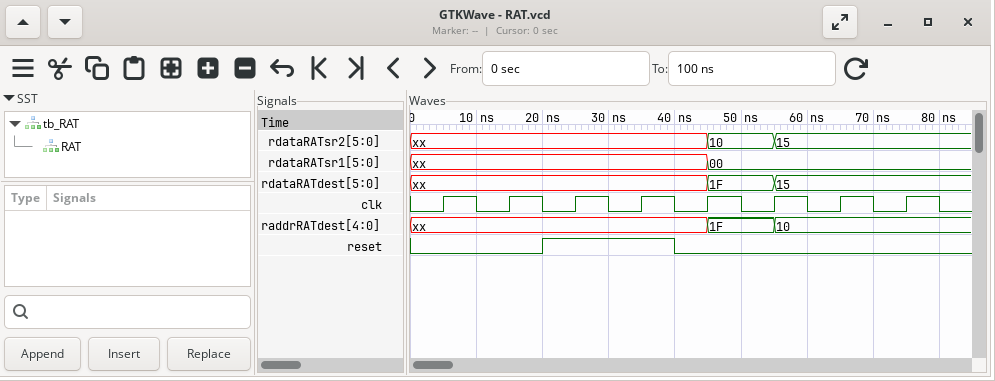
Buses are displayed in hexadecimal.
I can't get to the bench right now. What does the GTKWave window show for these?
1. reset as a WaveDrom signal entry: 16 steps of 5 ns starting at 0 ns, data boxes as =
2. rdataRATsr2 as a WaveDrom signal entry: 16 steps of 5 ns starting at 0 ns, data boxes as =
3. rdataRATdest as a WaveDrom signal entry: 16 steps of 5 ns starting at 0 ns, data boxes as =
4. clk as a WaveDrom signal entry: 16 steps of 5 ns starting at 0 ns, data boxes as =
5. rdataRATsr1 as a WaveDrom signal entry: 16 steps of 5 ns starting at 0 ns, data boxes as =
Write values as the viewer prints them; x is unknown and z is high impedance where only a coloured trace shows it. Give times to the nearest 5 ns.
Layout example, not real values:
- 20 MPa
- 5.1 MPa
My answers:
- {name: 'reset', wave: '0...1...0.......'}
- {name: 'rdataRATsr2', wave: 'x........=.=....', data: '10 15'}
- {name: 'rdataRATdest', wave: 'x........=.=....', data: '1F 15'}
- {name: 'clk', wave: '0101010101010101'}
- {name: 'rdataRATsr1', wave: 'x........=......', data: '00'}
